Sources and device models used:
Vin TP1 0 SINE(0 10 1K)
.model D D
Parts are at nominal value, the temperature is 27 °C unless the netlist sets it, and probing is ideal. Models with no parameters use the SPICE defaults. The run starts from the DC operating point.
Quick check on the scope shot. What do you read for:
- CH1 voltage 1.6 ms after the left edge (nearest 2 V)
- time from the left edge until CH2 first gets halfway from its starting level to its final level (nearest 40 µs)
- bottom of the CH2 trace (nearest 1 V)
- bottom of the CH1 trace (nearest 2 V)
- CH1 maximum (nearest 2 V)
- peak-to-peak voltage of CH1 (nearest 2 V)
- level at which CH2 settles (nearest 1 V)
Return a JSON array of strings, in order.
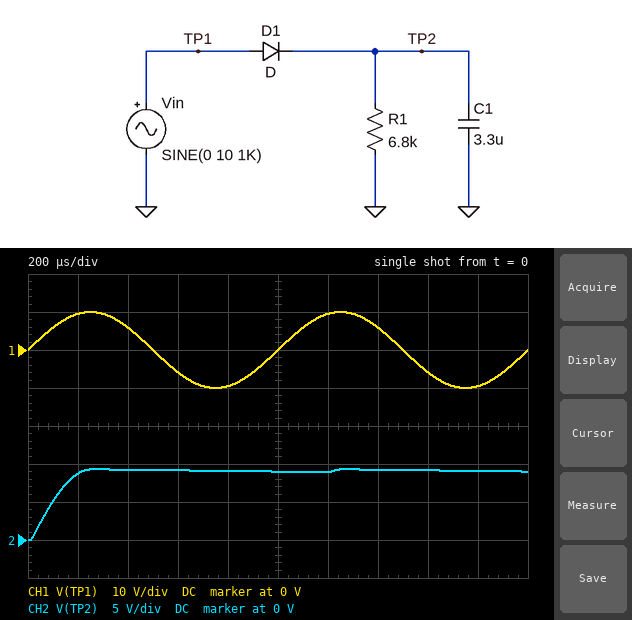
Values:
["-6 V", "80 µs", "0 V", "-10 V", "10 V", "20 V", "9 V"]
